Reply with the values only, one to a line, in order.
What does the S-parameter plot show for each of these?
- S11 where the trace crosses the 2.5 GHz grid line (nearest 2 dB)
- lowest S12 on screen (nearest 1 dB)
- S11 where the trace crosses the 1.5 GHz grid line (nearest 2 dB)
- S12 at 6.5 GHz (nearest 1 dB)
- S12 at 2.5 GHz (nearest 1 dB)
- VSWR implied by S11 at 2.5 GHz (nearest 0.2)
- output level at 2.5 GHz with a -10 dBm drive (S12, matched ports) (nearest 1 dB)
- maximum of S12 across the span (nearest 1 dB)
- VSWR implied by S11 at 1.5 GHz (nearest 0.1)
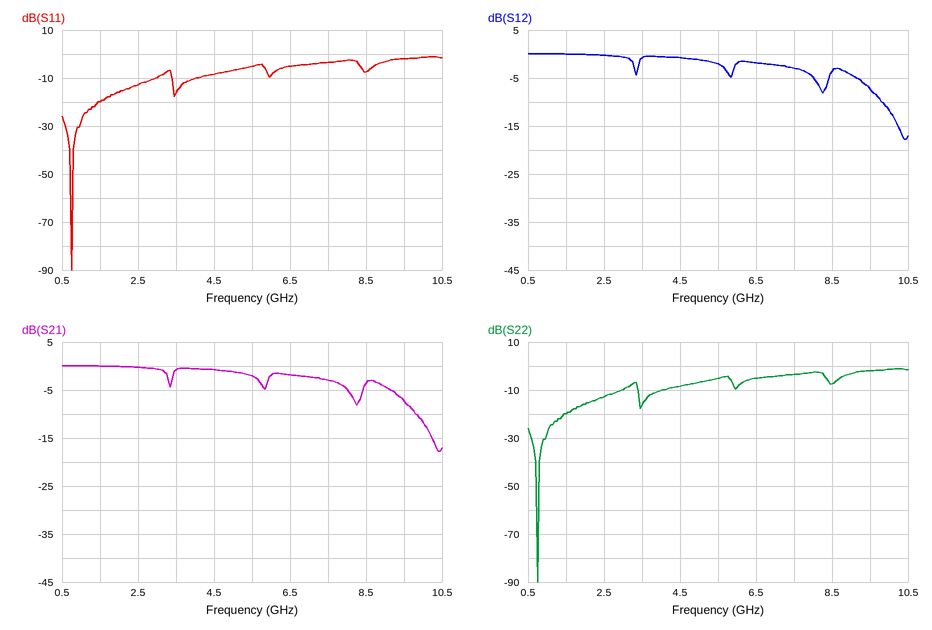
-12 dB
-18 dB
-20 dB
-2 dB
0 dB
1.6
-10 dBm
0 dB
1.2
